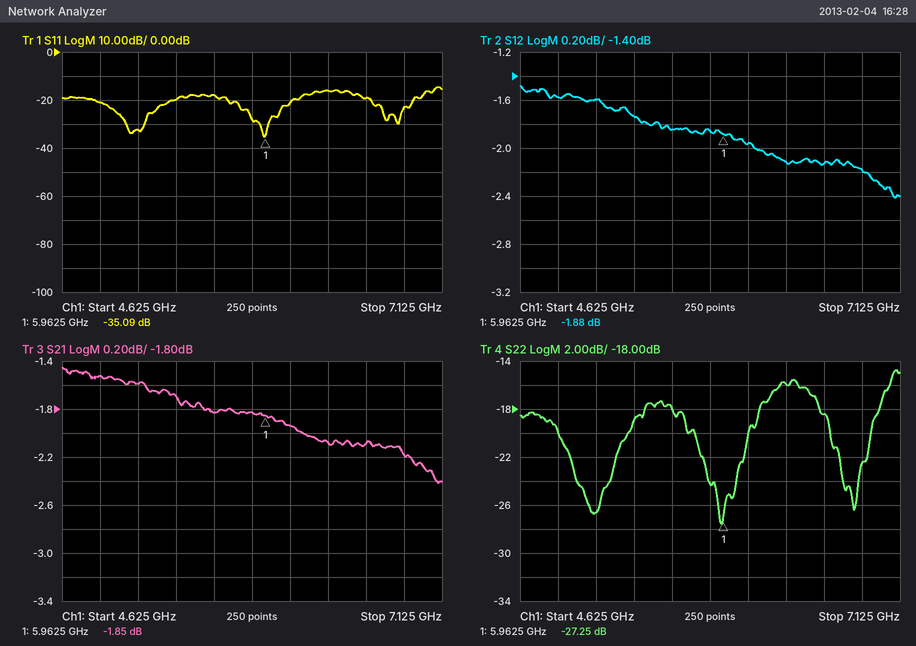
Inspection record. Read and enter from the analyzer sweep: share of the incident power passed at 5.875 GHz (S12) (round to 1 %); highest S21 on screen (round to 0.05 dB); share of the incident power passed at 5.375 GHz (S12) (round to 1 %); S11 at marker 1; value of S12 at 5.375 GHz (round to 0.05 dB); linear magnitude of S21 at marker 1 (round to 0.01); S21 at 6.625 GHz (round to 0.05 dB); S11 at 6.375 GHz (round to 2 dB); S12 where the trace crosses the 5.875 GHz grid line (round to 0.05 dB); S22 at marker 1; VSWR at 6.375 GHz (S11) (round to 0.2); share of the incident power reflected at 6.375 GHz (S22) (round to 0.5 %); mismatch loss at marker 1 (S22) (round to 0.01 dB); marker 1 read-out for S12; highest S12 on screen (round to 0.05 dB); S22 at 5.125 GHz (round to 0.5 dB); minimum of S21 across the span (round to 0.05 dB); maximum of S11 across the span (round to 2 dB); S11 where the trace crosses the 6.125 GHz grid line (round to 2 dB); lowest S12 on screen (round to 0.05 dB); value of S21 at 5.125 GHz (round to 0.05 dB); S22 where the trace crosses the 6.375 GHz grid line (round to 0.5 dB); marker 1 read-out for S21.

65 %
-1.45 dB
67 %
-35.09 dB
-1.75 dB
0.81
-2.10 dB
-16 dB
-1.85 dB
-27.25 dB
1.4
2.5 %
0.01 dB
-1.88 dB
-1.50 dB
-26.5 dB
-2.40 dB
-14 dB
-22 dB
-2.40 dB
-1.60 dB
-16.0 dB
-1.85 dB
